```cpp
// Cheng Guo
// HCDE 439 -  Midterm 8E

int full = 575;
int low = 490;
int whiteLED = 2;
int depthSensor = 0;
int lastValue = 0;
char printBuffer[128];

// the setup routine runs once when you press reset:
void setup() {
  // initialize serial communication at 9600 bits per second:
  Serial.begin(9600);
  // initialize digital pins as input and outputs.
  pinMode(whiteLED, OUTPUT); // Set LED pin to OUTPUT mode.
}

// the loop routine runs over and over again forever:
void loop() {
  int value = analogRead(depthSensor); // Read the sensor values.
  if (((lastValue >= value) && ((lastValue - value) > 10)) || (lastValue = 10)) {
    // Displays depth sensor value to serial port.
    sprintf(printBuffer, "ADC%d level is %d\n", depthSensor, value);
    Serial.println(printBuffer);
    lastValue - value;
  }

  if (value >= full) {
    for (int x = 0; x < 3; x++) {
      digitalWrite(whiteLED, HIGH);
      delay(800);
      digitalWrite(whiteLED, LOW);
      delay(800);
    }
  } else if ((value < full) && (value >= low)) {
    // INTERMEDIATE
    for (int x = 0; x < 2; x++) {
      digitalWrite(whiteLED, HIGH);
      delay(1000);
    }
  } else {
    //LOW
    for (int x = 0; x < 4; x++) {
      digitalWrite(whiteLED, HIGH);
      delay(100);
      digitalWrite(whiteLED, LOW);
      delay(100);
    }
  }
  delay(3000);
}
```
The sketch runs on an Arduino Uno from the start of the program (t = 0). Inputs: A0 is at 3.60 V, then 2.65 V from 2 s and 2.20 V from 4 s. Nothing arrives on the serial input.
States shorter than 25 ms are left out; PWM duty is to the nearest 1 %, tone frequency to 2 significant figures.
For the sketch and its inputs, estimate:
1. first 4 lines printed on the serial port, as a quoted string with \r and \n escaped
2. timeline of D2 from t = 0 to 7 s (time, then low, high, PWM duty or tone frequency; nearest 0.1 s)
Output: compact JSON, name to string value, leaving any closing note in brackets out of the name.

{"first 4 lines printed on the serial port, as a quoted string with \\r and \\n escaped": "\"ADC0 level is 737\\n\\r\\nADC0 level is 450\\n\\r\\n\"", "timeline of D2 from t = 0 to 7 s": "0 s high; 0.8 s low; 1.6 s high; 2.4 s low; 3.2 s high; 4 s low"}
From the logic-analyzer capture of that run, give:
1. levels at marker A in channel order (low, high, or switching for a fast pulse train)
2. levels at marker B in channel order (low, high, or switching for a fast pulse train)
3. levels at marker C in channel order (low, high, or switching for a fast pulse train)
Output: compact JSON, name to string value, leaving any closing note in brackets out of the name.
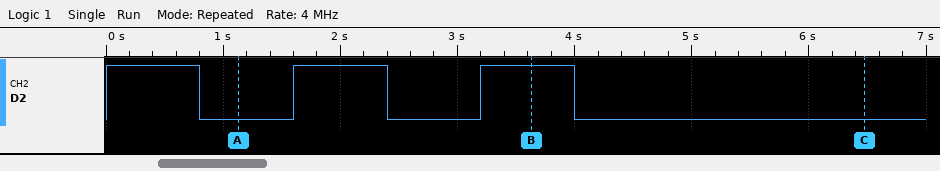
{"levels at marker A in channel order": "D2 low", "levels at marker B in channel order": "D2 high", "levels at marker C in channel order": "D2 low"}
